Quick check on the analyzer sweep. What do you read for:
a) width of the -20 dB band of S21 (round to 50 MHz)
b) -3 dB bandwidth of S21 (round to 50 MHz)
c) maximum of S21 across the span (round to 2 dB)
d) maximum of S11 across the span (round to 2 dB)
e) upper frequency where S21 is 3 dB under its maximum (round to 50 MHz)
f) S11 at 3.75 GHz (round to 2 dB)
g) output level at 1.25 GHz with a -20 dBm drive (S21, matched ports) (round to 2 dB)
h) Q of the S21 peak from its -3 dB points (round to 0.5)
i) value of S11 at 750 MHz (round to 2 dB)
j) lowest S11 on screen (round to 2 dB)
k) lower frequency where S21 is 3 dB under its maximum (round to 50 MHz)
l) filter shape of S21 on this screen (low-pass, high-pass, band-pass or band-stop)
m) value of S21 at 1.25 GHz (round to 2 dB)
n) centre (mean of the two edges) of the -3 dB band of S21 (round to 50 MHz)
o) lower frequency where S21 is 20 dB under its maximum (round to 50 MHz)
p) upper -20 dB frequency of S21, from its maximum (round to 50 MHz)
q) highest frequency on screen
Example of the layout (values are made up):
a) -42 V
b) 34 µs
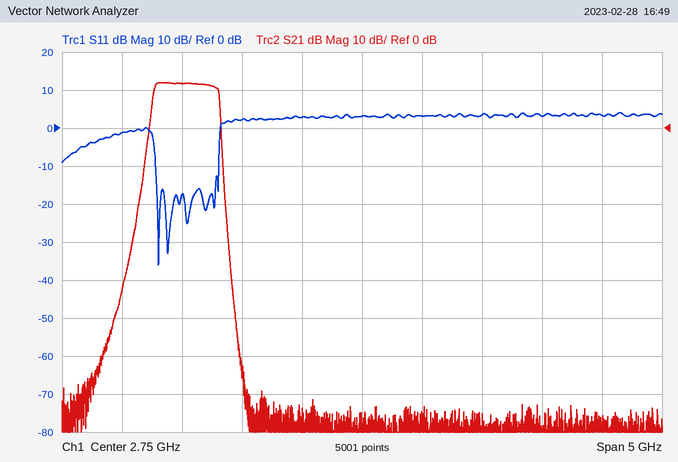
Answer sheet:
a) 650 MHz
b) 550 MHz
c) 12 dB
d) 4 dB
e) 1.55 GHz
f) 4 dB
g) -8 dBm
h) 2.5
i) -2 dB
j) -36 dB
k) 1.00 GHz
l) band-pass
m) 12 dB
n) 1.30 GHz
o) 950 MHz
p) 1.60 GHz
q) 5.25 GHz
